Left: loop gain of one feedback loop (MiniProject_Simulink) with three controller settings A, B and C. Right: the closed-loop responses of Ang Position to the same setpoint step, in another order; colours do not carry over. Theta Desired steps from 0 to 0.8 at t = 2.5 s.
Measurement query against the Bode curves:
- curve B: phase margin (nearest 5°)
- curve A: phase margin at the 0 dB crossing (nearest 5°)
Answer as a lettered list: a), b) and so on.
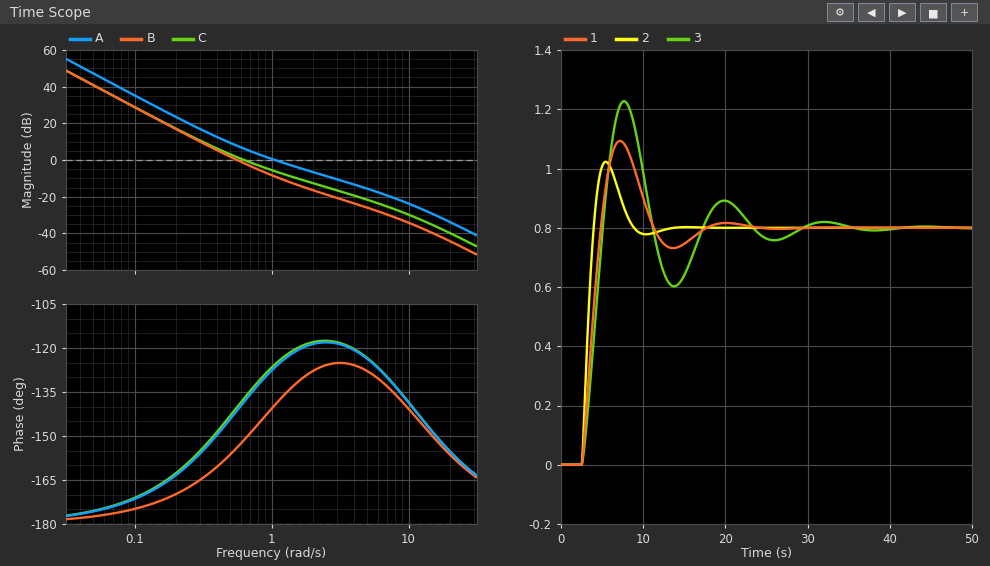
a) 25°
b) 55°
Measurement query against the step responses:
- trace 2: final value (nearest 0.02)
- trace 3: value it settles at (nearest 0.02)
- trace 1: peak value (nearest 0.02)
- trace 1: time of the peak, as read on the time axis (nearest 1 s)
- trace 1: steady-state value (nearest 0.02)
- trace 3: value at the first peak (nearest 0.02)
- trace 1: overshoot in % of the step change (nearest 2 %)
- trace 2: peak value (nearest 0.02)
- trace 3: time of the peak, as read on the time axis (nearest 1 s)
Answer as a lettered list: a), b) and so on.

a) 0.80
b) 0.80
c) 1.10
d) 7 s
e) 0.80
f) 1.22
g) 36 %
h) 1.02
i) 8 s
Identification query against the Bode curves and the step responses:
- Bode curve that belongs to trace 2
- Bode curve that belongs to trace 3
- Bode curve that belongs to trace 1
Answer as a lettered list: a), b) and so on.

a) A
b) B
c) C
